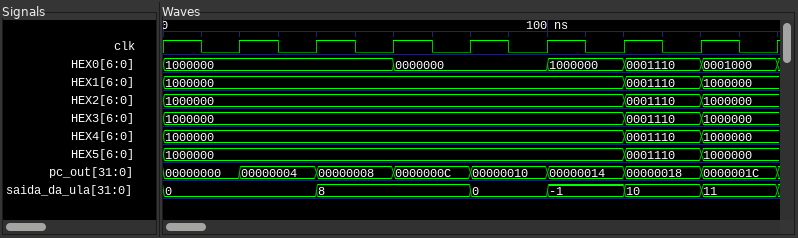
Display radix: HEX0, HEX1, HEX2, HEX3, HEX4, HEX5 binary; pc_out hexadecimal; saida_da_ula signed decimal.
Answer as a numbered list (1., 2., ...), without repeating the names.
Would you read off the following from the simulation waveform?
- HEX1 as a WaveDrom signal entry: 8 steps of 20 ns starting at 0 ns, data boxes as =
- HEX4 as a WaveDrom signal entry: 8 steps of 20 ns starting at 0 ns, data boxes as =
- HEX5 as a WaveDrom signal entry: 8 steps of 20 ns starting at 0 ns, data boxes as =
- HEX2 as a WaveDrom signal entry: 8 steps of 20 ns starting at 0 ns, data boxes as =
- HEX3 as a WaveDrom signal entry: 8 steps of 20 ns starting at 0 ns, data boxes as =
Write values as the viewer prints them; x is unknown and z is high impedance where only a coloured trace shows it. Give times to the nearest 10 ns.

1. {name: 'HEX1', wave: '=.....==', data: '1000000 0001110 1000000'}
2. {name: 'HEX4', wave: '=.....==', data: '1000000 0001110 1000000'}
3. {name: 'HEX5', wave: '=.....==', data: '1000000 0001110 1000000'}
4. {name: 'HEX2', wave: '=.....==', data: '1000000 0001110 1000000'}
5. {name: 'HEX3', wave: '=.....==', data: '1000000 0001110 1000000'}
